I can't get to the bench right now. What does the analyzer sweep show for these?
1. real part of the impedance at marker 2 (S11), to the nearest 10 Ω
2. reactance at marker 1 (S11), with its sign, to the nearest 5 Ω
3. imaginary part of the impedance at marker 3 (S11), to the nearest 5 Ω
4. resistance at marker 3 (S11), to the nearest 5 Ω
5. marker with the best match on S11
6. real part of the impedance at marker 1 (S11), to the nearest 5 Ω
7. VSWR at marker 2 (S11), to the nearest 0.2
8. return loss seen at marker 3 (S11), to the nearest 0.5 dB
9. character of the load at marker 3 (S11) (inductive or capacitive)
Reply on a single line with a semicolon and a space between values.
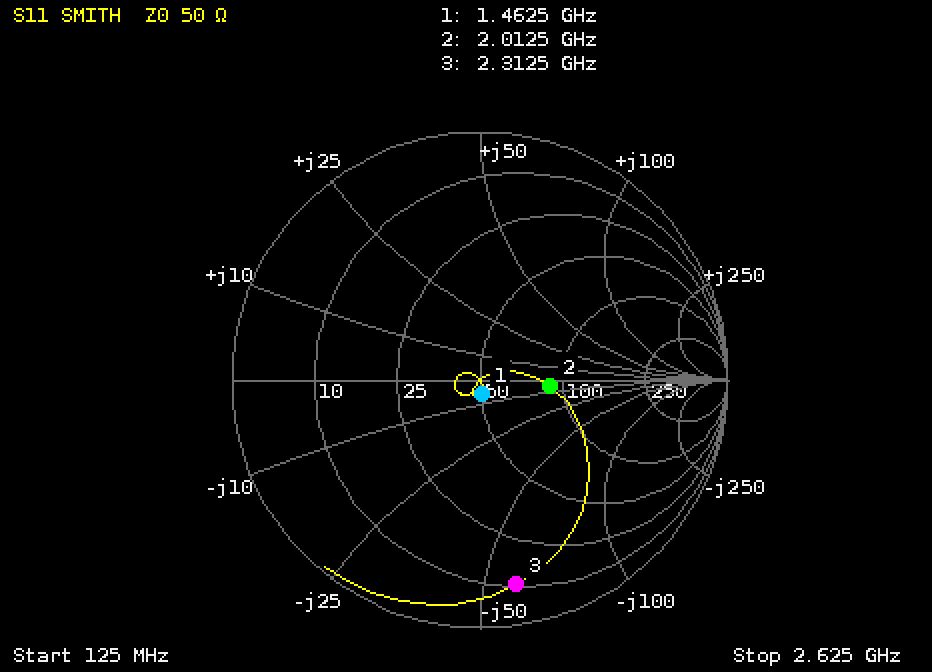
90 Ω; -5 Ω; -60 Ω; 10 Ω; marker 1; 50 Ω; 1.8; 1.5 dB; capacitive
